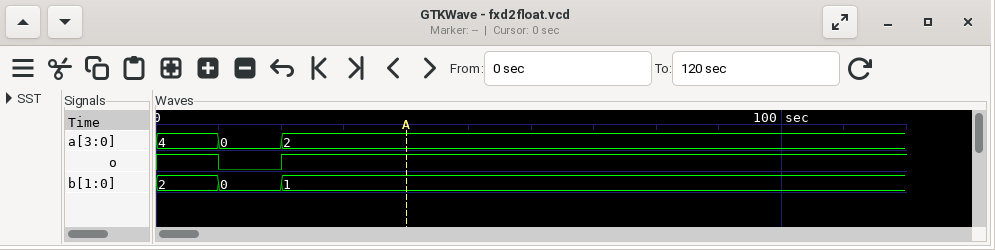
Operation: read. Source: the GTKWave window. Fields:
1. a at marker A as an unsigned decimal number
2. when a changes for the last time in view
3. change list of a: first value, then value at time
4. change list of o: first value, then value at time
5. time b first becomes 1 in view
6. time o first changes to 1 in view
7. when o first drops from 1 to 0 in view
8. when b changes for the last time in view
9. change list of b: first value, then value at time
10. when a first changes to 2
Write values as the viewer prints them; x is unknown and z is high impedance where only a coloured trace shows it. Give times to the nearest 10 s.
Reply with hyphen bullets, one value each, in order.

- 2
- 20 s
- 4, 0 at 10 s, 2 at 20 s
- 1, 0 at 10 s, 1 at 20 s
- 20 s
- 20 s
- 10 s
- 20 s
- 2, 0 at 10 s, 1 at 20 s
- 20 s
